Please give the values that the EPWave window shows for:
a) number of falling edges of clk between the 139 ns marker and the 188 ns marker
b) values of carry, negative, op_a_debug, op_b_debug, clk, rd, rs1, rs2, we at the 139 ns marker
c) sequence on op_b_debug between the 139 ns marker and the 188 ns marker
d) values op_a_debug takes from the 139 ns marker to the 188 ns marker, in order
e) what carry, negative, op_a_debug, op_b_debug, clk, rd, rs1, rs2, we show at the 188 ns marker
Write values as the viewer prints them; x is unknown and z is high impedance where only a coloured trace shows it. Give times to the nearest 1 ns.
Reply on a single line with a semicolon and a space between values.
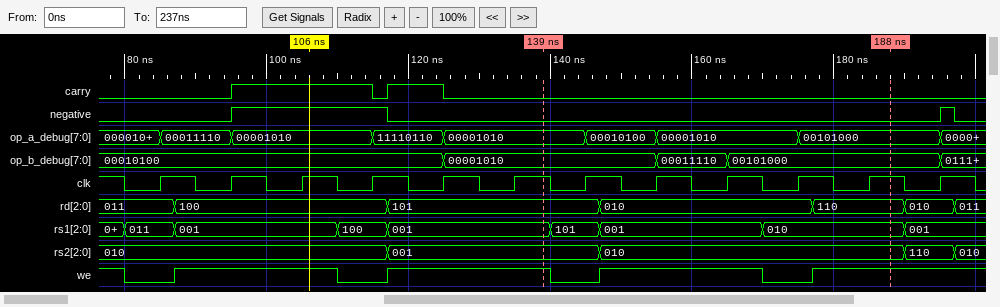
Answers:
5; carry=0, negative=0, op_a_debug=00001010, op_b_debug=00001010, clk=1, rd=101, rs1=001, rs2=001, we=1; 00001010, 00011110, 00101000; 00001010, 00010100, 00001010, 00101000; carry=0, negative=0, op_a_debug=00101000, op_b_debug=00101000, clk=1, rd=110, rs1=010, rs2=010, we=1
